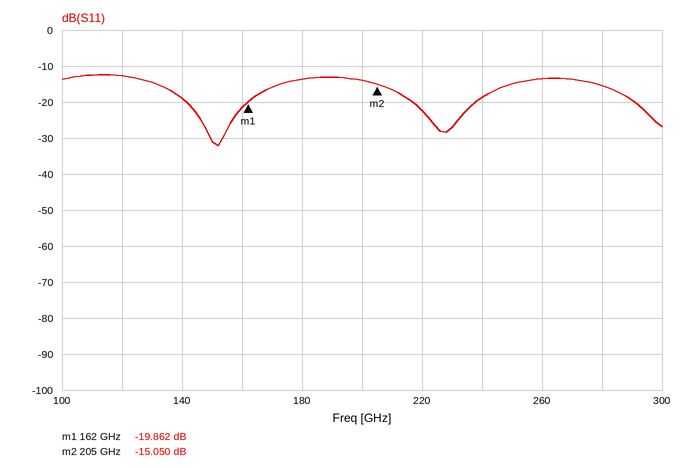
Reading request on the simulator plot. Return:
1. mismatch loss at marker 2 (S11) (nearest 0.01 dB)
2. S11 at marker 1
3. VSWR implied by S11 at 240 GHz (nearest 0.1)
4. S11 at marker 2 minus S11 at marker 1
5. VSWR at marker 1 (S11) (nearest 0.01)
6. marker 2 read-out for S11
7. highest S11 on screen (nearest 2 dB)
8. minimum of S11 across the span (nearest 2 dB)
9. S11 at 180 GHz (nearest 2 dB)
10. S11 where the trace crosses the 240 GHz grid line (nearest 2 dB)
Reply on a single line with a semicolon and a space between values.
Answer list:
0.14 dB; -19.862 dB; 1.3; 4.812 dB; 1.23; -15.050 dB; -12 dB; -32 dB; -14 dB; -18 dB
